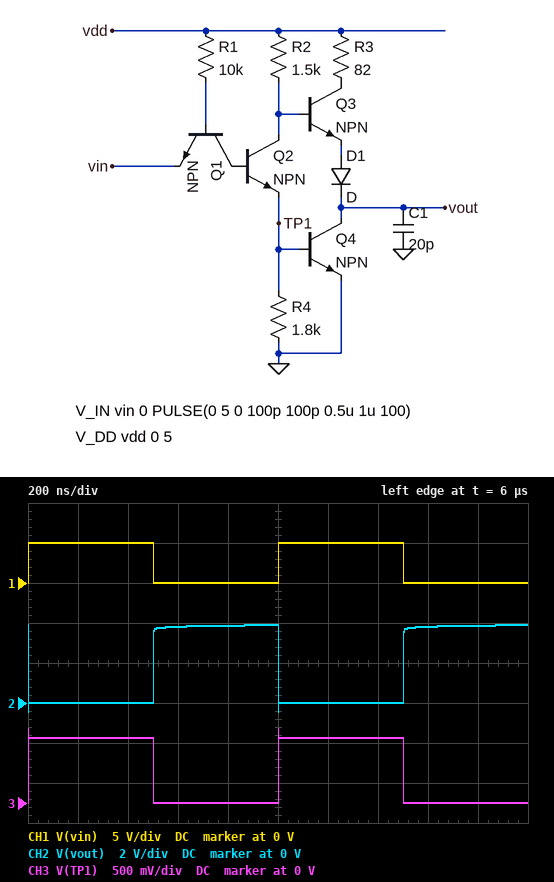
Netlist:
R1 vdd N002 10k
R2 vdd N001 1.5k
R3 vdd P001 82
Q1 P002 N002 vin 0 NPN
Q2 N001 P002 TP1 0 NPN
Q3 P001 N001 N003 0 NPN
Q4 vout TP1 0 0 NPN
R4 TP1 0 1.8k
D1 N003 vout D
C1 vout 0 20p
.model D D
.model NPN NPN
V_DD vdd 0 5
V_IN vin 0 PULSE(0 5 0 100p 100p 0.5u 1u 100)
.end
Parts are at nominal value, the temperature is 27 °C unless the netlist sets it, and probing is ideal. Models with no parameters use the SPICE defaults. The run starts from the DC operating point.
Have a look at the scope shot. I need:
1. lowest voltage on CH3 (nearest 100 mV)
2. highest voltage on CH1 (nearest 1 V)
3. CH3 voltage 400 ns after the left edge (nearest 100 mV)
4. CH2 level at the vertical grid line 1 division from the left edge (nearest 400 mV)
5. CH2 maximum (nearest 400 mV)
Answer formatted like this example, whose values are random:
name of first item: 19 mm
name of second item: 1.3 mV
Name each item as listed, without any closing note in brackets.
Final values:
lowest voltage on CH3: 0 V
highest voltage on CH1: 5 V
CH3 voltage 400 ns after the left edge: 800 mV
CH2 level at the vertical grid line 1 division from the left edge: 0 V
CH2 maximum: 4.0 V
